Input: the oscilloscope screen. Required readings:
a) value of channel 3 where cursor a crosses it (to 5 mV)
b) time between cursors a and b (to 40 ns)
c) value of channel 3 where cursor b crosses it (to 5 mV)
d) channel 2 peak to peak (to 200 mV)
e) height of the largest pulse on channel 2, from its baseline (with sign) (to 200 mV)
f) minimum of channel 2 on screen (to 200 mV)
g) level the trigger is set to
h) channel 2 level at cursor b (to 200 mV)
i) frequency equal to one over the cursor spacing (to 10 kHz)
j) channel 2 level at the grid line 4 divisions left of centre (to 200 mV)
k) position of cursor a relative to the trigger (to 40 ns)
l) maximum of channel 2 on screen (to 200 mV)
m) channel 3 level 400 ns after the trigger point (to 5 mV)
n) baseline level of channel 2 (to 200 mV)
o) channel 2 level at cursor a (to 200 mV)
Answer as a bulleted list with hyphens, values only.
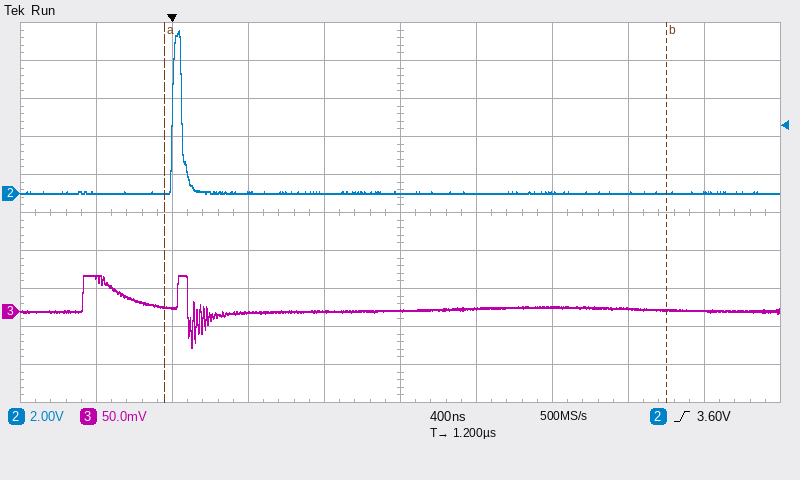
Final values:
- 5 mV
- 2.64 µs
- 0 mV
- 8.6 V
- +8.6 V
- 0.0 V
- 3.60 V
- 0.0 V
- 380 kHz
- 0.0 V
- -40 ns
- 8.6 V
- 0 mV
- 0.0 V
- 0.0 V
